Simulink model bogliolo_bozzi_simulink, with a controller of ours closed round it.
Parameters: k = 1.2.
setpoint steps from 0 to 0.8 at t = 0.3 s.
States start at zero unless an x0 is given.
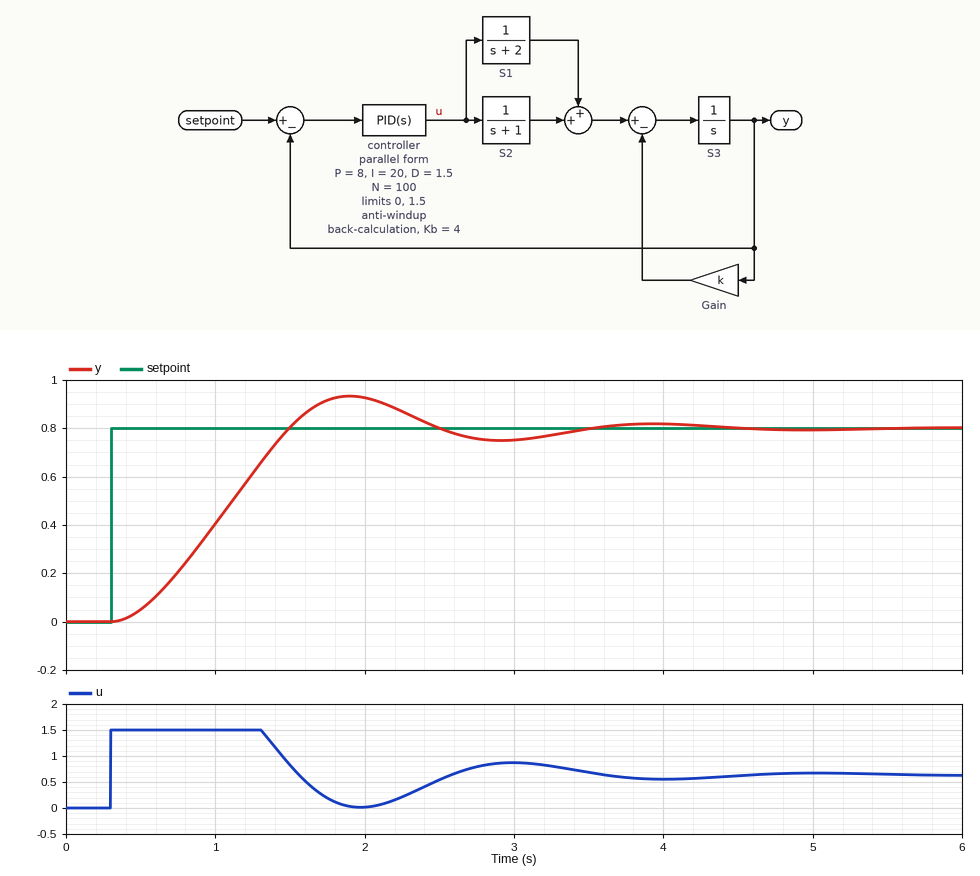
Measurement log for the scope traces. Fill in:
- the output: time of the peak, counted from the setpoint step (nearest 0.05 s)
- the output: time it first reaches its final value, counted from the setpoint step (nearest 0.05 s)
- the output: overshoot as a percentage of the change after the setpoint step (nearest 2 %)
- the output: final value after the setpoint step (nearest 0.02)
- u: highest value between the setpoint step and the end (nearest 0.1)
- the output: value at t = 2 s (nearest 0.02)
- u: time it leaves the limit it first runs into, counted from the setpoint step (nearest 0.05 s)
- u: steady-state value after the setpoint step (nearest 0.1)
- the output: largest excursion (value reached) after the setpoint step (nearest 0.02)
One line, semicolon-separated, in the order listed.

1.60 s; 1.20 s; 16 %; 0.80; 1.5; 0.92; 1.00 s; 0.6; 0.94
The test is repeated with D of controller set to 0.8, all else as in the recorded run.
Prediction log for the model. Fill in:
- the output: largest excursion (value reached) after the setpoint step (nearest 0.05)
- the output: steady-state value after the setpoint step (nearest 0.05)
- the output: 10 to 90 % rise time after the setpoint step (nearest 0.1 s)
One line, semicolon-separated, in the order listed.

0.90; 0.80; 0.8 s
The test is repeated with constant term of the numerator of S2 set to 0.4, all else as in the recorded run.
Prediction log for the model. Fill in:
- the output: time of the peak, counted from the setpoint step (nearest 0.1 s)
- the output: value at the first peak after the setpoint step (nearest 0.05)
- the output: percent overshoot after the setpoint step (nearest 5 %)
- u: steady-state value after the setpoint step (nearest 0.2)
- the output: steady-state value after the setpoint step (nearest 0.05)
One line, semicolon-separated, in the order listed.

2.4 s; 0.85; 10 %; 1.0; 0.80
